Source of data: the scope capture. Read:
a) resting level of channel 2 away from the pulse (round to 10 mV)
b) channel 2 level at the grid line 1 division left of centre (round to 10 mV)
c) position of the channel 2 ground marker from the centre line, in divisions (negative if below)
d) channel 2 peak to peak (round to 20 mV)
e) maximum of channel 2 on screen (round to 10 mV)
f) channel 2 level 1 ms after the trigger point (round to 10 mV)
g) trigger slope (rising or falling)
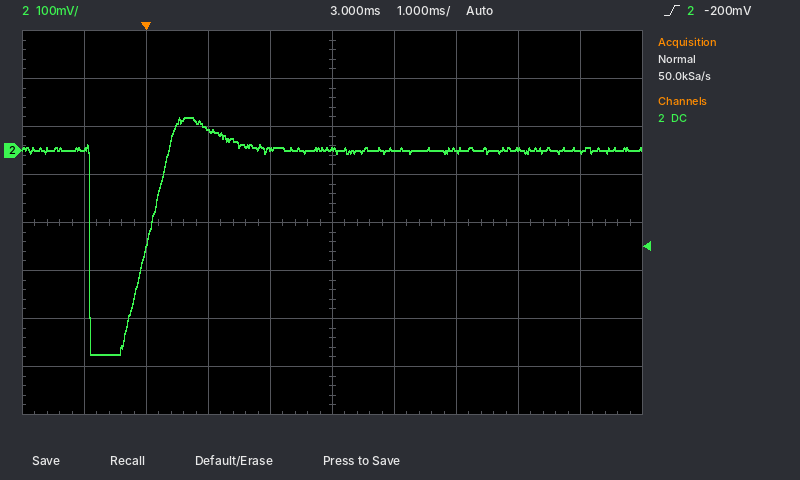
0 mV
0 mV
+1.5 div
500 mV
70 mV
40 mV
rising
